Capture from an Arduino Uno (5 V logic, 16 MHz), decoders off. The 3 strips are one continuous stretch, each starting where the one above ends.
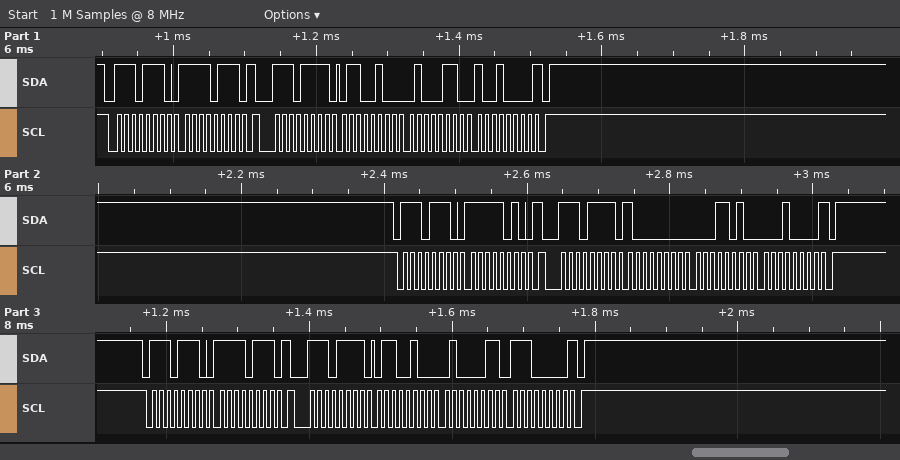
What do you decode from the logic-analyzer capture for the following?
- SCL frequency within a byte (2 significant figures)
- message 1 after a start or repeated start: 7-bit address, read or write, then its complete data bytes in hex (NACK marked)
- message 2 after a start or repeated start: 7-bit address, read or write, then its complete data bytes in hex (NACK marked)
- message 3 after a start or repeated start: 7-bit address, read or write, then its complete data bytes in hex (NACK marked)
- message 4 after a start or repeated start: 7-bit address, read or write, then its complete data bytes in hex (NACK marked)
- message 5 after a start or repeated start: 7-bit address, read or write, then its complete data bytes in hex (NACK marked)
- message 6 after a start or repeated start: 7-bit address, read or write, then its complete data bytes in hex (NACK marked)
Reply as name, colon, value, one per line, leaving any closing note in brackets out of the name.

SCL frequency within a byte: 100 kHz
message 1 after a start or repeated start: 7-bit address, read or write, then its complete data bytes in hex: 0x77 write: F7
message 2 after a start or repeated start: 7-bit address, read or write, then its complete data bytes in hex: 0x77 read: 64 46 90 NACK
message 3 after a start or repeated start: 7-bit address, read or write, then its complete data bytes in hex: 0x77 write: FA
message 4 after a start or repeated start: 7-bit address, read or write, then its complete data bytes in hex: 0x77 read: 80 1A 10 NACK
message 5 after a start or repeated start: 7-bit address, read or write, then its complete data bytes in hex: 0x77 write: F7
message 6 after a start or repeated start: 7-bit address, read or write, then its complete data bytes in hex: 0x77 read: 64 43 E0 NACK
